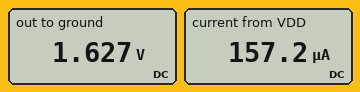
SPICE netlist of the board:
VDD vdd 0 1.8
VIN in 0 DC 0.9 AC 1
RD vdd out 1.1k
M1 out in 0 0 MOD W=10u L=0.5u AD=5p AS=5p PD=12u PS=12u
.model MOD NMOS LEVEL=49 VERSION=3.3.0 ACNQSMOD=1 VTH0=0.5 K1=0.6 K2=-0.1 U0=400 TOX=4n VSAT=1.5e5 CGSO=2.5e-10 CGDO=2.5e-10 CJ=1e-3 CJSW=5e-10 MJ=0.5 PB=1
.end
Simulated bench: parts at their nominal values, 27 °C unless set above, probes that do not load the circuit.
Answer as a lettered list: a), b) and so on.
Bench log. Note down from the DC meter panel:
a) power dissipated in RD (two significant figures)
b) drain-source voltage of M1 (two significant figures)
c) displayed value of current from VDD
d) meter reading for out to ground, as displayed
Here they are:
a) 27 µW
b) 1.6 V
c) 157.2 µA
d) 1.627 V
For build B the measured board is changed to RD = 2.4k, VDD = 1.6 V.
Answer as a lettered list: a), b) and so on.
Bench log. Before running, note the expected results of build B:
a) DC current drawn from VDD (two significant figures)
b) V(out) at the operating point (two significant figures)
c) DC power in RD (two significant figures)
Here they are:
a) 150 µA
b) 1.2 V
c) 57 µW
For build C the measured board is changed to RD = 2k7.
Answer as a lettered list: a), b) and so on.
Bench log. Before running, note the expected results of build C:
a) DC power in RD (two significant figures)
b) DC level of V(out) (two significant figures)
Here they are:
a) 65 µW
b) 1.4 V
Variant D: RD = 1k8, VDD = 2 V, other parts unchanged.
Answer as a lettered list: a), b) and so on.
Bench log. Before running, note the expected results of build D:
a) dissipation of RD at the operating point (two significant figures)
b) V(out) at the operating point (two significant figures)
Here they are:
a) 45 µW
b) 1.7 V
